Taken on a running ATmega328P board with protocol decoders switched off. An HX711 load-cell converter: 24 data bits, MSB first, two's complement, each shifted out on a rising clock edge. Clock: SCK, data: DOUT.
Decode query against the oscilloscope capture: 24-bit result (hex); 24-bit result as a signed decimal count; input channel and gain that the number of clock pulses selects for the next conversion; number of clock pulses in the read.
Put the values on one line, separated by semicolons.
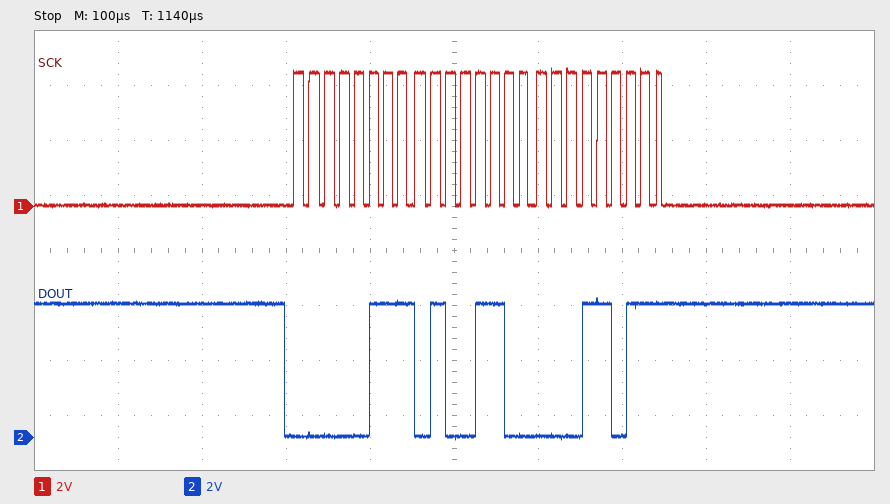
0x074C1B; 478235; channel A, gain 128; 25
